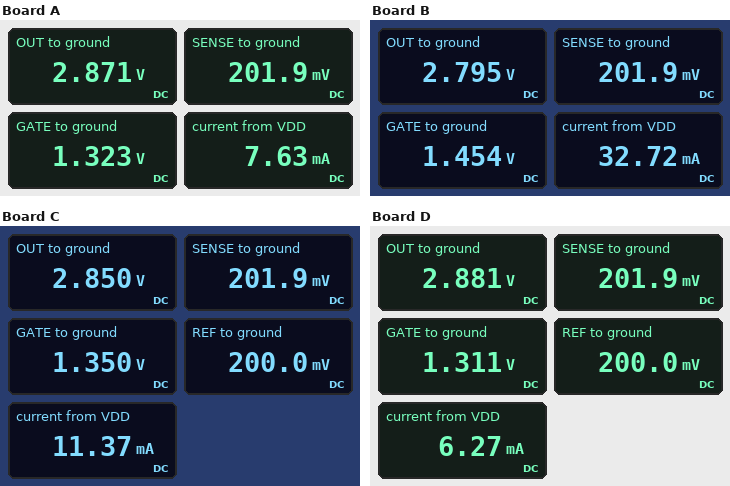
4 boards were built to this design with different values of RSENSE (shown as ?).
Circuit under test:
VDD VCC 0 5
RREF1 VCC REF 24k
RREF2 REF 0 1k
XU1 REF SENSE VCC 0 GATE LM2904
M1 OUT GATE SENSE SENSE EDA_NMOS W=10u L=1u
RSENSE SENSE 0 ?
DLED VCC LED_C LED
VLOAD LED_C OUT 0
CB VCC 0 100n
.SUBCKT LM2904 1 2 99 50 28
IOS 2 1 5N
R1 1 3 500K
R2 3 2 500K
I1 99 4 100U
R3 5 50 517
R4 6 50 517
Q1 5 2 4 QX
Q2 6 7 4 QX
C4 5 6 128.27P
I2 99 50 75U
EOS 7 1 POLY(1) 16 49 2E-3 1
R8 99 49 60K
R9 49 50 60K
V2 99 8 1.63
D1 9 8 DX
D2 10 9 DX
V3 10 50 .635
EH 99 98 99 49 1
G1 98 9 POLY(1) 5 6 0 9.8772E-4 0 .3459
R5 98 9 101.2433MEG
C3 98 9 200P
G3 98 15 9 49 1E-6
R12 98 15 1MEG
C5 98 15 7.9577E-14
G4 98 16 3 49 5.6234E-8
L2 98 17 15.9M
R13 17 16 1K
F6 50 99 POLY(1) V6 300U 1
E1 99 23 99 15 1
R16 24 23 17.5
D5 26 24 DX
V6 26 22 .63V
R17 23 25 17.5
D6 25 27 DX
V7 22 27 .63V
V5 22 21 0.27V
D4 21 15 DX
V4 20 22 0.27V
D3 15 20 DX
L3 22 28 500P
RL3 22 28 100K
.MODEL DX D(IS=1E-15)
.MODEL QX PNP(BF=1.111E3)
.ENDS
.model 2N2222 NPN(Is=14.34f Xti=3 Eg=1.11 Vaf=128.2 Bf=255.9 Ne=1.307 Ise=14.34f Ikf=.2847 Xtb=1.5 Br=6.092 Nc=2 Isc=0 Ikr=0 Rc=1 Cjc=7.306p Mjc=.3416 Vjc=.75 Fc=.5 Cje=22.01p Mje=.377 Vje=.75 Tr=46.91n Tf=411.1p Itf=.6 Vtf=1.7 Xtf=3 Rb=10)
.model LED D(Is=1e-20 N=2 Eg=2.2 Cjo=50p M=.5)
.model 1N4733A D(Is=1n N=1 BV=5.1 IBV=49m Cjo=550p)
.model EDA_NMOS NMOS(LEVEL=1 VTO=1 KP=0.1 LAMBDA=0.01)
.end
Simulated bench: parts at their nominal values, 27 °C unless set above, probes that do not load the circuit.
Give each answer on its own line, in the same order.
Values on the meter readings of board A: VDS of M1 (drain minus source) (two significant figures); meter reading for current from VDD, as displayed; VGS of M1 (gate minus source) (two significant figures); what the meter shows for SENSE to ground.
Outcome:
2.7 V
7.63 mA
1.1 V
201.9 mV
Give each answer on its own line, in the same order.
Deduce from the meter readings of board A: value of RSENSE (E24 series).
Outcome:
27 Ω
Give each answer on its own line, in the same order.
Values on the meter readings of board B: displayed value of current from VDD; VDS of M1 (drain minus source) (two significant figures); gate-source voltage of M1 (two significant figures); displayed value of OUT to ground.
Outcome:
32.72 mA
2.6 V
1.3 V
2.795 V
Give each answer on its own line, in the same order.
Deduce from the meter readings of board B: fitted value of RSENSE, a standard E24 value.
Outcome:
6.2 Ω
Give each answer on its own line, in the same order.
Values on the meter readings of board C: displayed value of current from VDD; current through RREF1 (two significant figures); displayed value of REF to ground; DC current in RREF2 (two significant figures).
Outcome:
11.37 mA
200 µA
200.0 mV
200 µA
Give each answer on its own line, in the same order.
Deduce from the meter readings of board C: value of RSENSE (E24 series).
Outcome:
18 Ω
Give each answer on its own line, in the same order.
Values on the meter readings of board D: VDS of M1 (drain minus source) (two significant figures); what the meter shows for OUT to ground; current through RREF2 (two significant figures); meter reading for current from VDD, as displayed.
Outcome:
2.7 V
2.881 V
200 µA
6.27 mA
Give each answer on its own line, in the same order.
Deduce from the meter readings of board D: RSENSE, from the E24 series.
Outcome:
33 Ω
